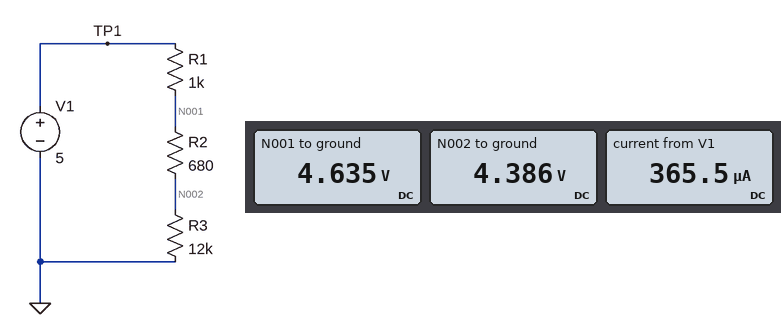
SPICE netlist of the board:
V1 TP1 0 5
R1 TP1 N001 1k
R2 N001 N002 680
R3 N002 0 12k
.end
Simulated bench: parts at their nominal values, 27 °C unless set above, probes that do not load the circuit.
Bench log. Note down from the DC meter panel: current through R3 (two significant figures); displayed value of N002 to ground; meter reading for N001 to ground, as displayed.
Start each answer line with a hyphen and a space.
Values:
- 370 µA
- 4.386 V
- 4.635 V
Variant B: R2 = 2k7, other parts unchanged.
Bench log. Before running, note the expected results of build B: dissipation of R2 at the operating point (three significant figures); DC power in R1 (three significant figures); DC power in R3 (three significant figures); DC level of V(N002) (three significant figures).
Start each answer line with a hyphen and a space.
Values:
- 274 µW
- 101 µW
- 1.22 mW
- 3.82 V
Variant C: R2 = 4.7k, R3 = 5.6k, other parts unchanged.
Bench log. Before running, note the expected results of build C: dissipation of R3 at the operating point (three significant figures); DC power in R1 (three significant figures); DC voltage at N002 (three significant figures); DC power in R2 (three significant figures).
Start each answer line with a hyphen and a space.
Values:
- 1.10 mW
- 196 µW
- 2.48 V
- 920 µW
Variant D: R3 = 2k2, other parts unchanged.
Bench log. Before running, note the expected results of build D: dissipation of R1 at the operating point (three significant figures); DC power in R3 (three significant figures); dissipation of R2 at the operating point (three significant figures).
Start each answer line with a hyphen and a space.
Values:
- 1.66 mW
- 3.65 mW
- 1.13 mW
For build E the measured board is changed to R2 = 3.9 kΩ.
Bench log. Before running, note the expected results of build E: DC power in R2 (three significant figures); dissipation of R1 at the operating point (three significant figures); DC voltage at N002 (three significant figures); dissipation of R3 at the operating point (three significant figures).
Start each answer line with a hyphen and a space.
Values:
- 341 µW
- 87.5 µW
- 3.55 V
- 1.05 mW
